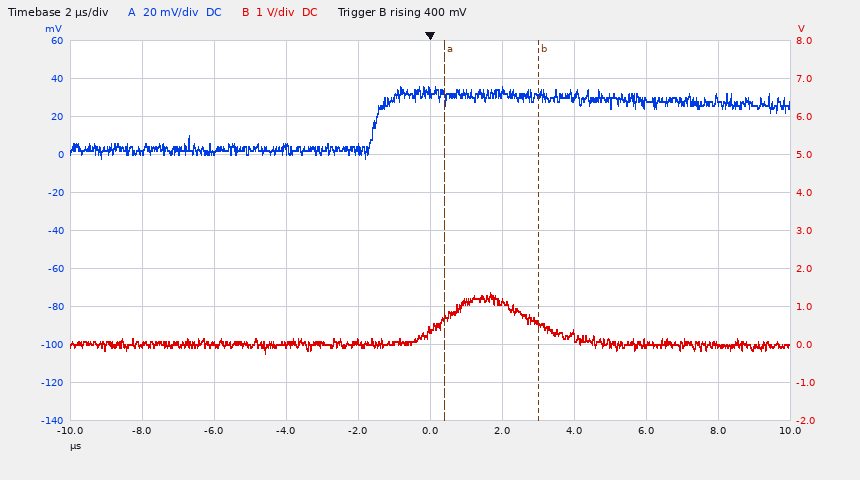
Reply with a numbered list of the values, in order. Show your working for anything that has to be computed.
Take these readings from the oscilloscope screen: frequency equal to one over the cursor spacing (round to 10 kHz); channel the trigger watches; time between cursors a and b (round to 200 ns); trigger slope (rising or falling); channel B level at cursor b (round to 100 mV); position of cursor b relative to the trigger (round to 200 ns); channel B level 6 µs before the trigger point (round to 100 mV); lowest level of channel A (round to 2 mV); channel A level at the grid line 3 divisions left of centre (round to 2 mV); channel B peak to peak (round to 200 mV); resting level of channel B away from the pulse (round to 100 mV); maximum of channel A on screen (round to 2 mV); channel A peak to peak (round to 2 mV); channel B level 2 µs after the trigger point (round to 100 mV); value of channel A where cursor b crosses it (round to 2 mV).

1. 1 / 2.6 µs ≈ 380 kHz
2. channel B
3. 2.6 µs
4. rising
5. 600 mV
6. +3.0 µs
7. 0.0 V
8. -2 mV
9. 2 mV
10. 1.6 V
11. 0.0 V
12. 36 mV
13. 36 mV − (-2 mV) = 38 mV
14. 1.1 V
15. 32 mV
